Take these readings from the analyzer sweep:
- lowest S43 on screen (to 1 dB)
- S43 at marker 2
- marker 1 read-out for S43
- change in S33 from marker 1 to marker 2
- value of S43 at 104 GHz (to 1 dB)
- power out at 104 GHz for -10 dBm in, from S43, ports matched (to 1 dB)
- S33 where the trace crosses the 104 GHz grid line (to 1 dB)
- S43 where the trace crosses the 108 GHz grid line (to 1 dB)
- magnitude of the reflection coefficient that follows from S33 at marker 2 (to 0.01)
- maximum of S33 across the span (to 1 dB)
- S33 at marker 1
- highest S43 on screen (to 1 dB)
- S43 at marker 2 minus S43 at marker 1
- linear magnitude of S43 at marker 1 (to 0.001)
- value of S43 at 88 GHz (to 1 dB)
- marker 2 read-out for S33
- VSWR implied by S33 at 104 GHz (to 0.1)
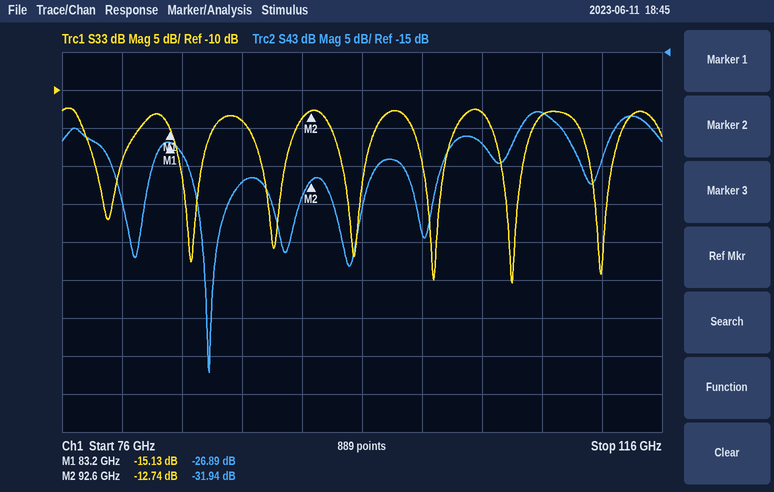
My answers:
-57 dB
-31.94 dB
-26.89 dB
2.39 dB
-27 dB
-37 dBm
-13 dB
-23 dB
0.23
-12 dB
-15.13 dB
-23 dB
-5.05 dB
0.045
-32 dB
-12.74 dB
1.6
